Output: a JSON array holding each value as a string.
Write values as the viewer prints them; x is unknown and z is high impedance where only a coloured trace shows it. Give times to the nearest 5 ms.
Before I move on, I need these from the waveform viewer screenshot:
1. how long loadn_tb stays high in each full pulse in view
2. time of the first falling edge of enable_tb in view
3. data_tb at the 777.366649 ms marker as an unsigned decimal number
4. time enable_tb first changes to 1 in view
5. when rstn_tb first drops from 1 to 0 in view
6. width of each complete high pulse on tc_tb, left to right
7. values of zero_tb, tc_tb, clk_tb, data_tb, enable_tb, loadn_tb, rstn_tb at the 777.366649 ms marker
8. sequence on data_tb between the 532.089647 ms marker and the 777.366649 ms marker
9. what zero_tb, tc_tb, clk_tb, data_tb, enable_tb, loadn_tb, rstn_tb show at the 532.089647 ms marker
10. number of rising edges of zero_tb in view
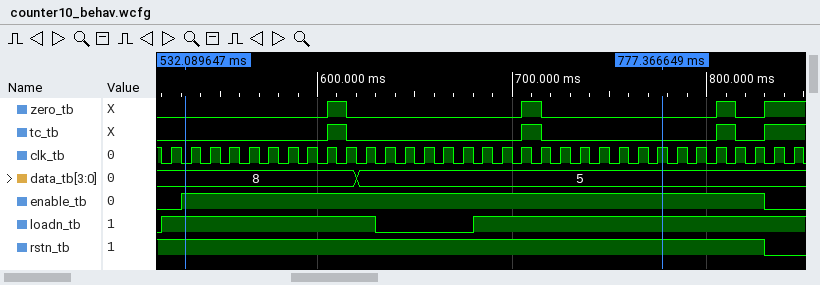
["110 ms", "830 ms", "5", "530 ms", "830 ms", "10 ms, 10 ms, 10 ms", "zero_tb=0, tc_tb=0, clk_tb=1, data_tb=5, enable_tb=1, loadn_tb=1, rstn_tb=1", "8, 5", "zero_tb=0, tc_tb=0, clk_tb=0, data_tb=8, enable_tb=1, loadn_tb=1, rstn_tb=1", "4"]
